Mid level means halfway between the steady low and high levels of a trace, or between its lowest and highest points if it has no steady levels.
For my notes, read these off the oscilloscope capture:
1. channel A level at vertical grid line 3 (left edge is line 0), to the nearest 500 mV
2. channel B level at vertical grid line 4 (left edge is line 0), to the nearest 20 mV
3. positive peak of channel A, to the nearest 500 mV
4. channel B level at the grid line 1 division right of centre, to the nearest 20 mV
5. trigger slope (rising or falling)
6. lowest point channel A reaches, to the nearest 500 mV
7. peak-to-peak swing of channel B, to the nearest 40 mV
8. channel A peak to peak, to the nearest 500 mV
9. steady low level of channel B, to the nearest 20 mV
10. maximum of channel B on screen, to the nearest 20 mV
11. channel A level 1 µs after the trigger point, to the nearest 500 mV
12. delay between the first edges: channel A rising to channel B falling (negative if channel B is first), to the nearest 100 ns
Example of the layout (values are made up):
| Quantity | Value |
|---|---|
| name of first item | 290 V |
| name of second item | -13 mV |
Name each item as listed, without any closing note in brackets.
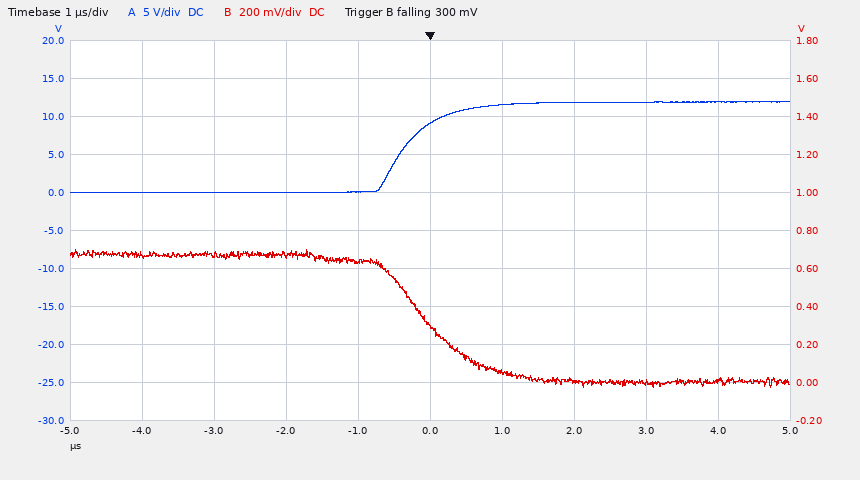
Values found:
| Quantity | Value |
|---|---|
| channel A level at vertical grid line 3 (left edge is line 0), to the nearest 500 mV | 0.0 V |
| channel B level at vertical grid line 4 (left edge is line 0), to the nearest 20 mV | 640 mV |
| positive peak of channel A, to the nearest 500 mV | 12.0 V |
| channel B level at the grid line 1 division right of centre, to the nearest 20 mV | 60 mV |
| trigger slope | falling |
| lowest point channel A reaches, to the nearest 500 mV | 0.0 V |
| peak-to-peak swing of channel B, to the nearest 40 mV | 720 mV |
| channel A peak to peak, to the nearest 500 mV | 12.0 V |
| steady low level of channel B, to the nearest 20 mV | 0 mV |
| maximum of channel B on screen, to the nearest 20 mV | 700 mV |
| channel A level 1 µs after the trigger point, to the nearest 500 mV | 11.5 V |
| delay between the first edges: channel A rising to channel B falling (negative if channel B is first), to the nearest 100 ns | +300 ns |
